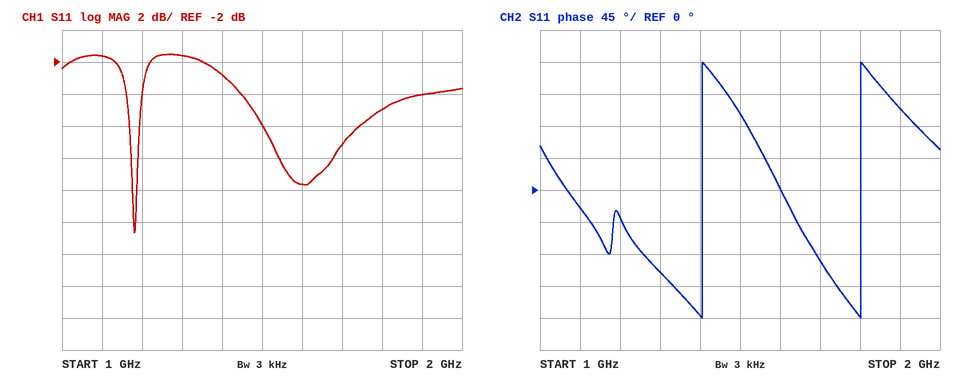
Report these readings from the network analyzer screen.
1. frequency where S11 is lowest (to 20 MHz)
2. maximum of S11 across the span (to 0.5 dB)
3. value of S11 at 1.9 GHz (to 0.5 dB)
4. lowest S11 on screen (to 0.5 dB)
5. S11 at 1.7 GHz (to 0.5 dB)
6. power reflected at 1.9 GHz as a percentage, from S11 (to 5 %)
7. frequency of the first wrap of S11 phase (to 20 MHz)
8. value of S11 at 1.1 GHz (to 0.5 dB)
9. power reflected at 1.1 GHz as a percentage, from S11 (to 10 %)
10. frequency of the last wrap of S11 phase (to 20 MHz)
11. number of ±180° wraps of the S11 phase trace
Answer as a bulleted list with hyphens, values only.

- 1.18 GHz
- -1.5 dB
- -4.0 dB
- -12.5 dB
- -7.0 dB
- 40 %
- 1.40 GHz
- -1.5 dB
- 70 %
- 1.80 GHz
- 2
